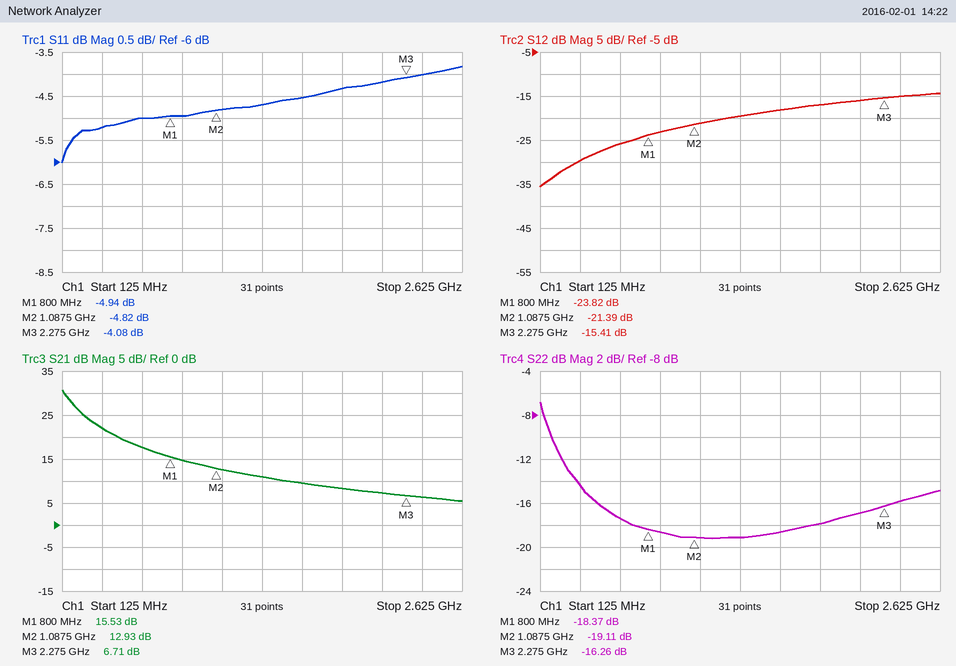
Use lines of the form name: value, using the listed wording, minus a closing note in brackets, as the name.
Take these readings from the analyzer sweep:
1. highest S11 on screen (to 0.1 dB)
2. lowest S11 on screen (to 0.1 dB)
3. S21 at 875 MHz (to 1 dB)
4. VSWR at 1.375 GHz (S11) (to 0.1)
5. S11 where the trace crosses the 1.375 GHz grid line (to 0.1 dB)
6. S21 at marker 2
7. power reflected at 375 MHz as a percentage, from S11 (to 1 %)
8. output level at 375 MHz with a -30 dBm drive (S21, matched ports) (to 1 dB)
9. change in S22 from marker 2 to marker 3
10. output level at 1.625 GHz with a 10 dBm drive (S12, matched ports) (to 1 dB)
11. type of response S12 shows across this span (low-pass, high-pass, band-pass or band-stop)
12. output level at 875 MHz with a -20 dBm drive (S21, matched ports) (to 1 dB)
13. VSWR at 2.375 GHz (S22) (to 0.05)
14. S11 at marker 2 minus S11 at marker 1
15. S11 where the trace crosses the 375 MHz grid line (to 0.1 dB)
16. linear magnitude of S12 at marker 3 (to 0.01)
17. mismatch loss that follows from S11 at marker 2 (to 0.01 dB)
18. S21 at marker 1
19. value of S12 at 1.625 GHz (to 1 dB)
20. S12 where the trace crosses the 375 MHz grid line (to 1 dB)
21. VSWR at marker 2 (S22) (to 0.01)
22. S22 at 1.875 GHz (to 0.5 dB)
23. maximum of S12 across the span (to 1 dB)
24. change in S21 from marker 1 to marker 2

highest S11 on screen: -3.8 dB
lowest S11 on screen: -6.0 dB
S21 at 875 MHz: 15 dB
VSWR at 1.375 GHz (S11): 3.8
S11 where the trace crosses the 1.375 GHz grid line: -4.7 dB
S21 at marker 2: 12.93 dB
power reflected at 375 MHz as a percentage, from S11: 30 %
output level at 375 MHz with a -30 dBm drive (S21, matched ports): -8 dBm
change in S22 from marker 2 to marker 3: 2.85 dB
output level at 1.625 GHz with a 10 dBm drive (S12, matched ports): -8 dBm
type of response S12 shows across this span: high-pass
output level at 875 MHz with a -20 dBm drive (S21, matched ports): -5 dBm
VSWR at 2.375 GHz (S22): 1.40
S11 at marker 2 minus S11 at marker 1: 0.12 dB
S11 where the trace crosses the 375 MHz grid line: -5.2 dB
linear magnitude of S12 at marker 3: 0.17
mismatch loss that follows from S11 at marker 2: 1.74 dB
S21 at marker 1: 15.53 dB
value of S12 at 1.625 GHz: -18 dB
S12 where the trace crosses the 375 MHz grid line: -30 dB
VSWR at marker 2 (S22): 1.25
S22 at 1.875 GHz: -18.0 dB
maximum of S12 across the span: -14 dB
change in S21 from marker 1 to marker 2: -2.60 dB
